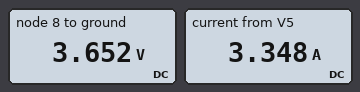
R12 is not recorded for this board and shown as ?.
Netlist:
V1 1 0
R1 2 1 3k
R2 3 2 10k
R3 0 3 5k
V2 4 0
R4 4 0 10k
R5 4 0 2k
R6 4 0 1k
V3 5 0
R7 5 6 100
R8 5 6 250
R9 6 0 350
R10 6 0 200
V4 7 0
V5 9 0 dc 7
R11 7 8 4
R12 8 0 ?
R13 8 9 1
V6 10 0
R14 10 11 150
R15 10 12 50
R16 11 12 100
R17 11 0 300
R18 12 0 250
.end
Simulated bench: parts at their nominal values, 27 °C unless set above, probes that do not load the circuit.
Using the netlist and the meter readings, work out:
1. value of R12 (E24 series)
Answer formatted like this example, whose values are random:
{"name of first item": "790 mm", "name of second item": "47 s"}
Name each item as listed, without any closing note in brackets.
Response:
{"value of R12": "1.5 Ω"}
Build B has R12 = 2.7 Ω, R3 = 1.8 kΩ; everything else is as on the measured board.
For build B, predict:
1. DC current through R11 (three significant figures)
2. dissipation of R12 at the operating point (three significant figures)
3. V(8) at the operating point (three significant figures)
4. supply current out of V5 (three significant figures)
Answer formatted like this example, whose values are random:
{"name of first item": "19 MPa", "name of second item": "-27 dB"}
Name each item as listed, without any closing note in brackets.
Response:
{"DC current through R11": "1.08 A", "dissipation of R12 at the operating point": "6.91 W", "V(8) at the operating point": "4.32 V", "supply current out of V5": "2.68 A"}
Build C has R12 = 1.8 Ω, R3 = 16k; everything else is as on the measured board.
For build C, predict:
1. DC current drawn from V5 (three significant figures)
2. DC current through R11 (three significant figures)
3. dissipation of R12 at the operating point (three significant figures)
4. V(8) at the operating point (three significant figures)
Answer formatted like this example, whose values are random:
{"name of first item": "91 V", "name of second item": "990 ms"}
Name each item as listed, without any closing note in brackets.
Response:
{"DC current drawn from V5": "3.12 A", "DC current through R11": "969 mA", "dissipation of R12 at the operating point": "8.35 W", "V(8) at the operating point": "3.88 V"}
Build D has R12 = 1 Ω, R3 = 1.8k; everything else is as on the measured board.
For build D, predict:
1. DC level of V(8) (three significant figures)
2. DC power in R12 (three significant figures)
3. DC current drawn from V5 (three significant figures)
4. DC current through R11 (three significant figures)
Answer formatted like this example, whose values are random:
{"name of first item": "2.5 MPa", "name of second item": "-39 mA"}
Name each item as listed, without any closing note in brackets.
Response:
{"DC level of V(8)": "3.11 V", "DC power in R12": "9.68 W", "DC current drawn from V5": "3.89 A", "DC current through R11": "778 mA"}
